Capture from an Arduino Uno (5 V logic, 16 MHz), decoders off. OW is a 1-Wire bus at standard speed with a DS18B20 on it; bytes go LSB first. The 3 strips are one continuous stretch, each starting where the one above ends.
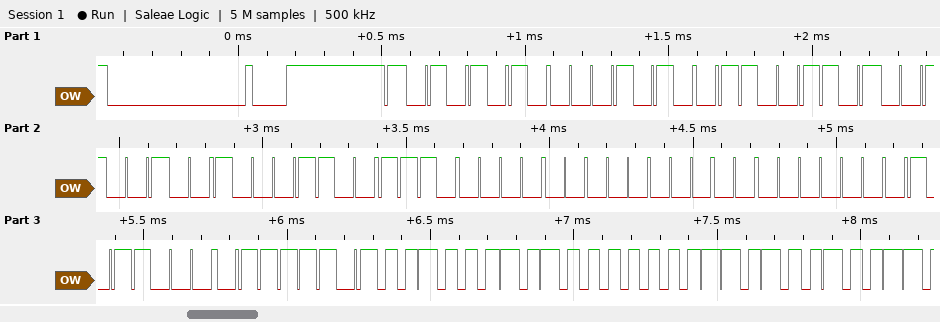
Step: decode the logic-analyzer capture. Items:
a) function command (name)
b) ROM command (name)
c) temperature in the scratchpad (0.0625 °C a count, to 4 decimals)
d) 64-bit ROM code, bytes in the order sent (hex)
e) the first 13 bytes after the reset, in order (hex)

Read Scratchpad
Match ROM
20.2500 °C
28 B3 24 31 07 00 00 1A
55 28 B3 24 31 07 00 00 1A BE 44 01 4B
